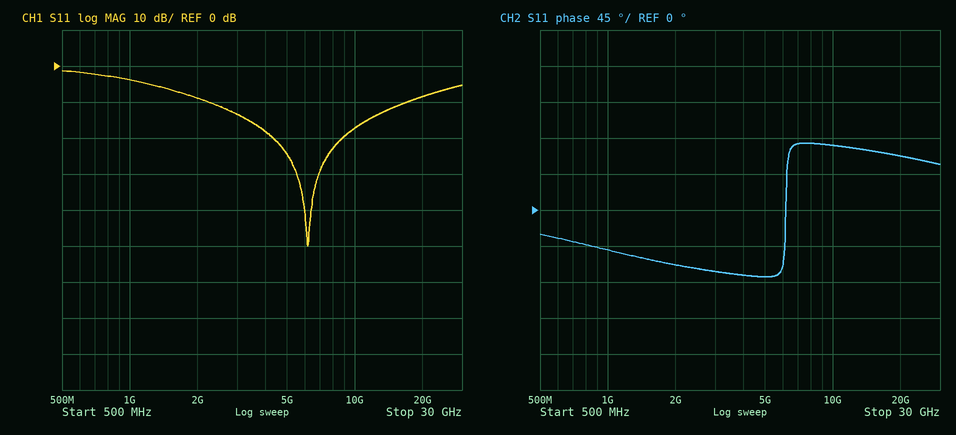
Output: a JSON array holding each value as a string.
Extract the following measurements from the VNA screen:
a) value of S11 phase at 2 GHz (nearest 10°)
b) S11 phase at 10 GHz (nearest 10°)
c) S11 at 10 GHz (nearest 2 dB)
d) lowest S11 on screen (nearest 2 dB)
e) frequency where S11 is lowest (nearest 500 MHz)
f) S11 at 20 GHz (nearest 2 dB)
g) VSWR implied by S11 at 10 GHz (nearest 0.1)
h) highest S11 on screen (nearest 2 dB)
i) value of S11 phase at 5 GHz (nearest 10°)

["-70°", "80°", "-18 dB", "-50 dB", "6.0 GHz", "-8 dB", "1.3", "-2 dB", "-80°"]
